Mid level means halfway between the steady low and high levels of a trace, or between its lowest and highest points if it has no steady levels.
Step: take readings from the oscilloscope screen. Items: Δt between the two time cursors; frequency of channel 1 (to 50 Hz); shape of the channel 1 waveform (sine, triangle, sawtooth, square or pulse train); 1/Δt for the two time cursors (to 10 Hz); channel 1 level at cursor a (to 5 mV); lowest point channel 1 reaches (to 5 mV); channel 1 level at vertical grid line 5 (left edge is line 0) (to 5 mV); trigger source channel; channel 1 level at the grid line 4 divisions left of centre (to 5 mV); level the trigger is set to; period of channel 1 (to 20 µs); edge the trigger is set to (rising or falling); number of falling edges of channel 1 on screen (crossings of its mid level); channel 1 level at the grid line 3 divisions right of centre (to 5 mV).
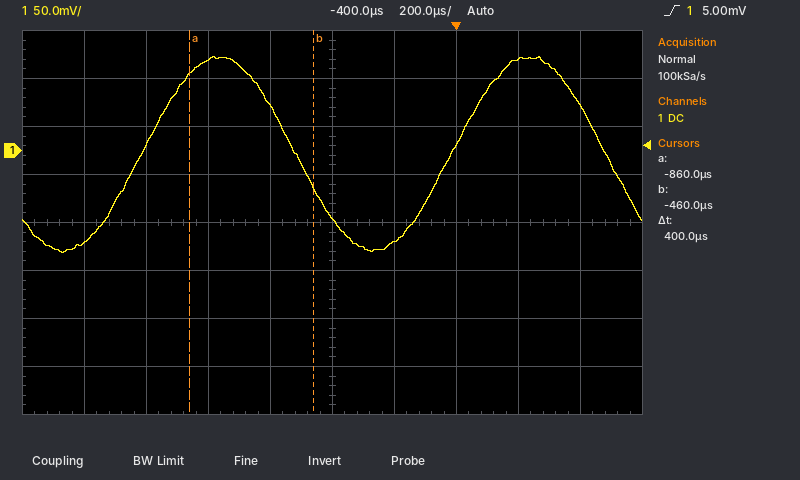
400 µs
1.00 kHz
sine
2.50 kHz
80 mV
-105 mV
-70 mV
channel 1
-95 mV
5.00 mV
1.00 ms
rising
2
95 mV
